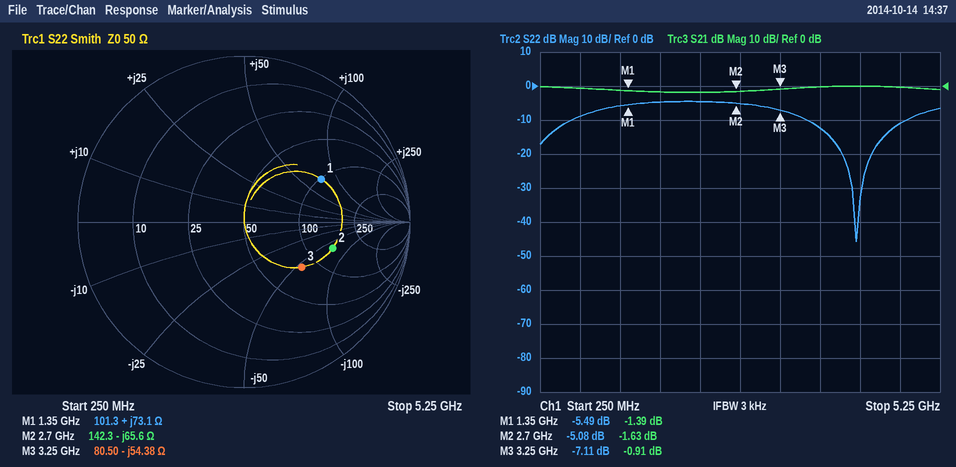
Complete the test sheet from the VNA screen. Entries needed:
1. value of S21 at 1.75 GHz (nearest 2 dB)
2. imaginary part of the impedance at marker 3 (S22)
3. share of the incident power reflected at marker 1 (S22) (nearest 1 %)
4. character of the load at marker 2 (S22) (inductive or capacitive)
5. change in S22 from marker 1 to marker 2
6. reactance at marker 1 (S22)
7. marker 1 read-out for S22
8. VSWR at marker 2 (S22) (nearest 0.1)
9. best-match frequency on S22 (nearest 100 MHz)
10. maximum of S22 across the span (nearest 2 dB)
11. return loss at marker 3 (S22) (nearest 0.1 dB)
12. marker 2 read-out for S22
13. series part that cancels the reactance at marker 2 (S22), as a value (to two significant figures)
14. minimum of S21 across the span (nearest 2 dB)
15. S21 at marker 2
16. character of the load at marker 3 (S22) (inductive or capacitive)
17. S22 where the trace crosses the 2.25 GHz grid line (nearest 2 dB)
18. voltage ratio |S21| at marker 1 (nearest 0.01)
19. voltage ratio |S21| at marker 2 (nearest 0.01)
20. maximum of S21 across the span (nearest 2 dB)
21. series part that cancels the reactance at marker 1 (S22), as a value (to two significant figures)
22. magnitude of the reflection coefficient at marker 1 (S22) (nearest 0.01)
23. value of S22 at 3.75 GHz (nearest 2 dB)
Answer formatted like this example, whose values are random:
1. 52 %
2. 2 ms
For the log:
1. -2 dB
2. -54.38 Ω
3. 28 %
4. capacitive
5. 0.41 dB
6. +73.1 Ω
7. -5.49 dB
8. 3.5
9. 4.2 GHz
10. -4 dB
11. 7.1 dB
12. -5.08 dB
13. 3.9 nH
14. -2 dB
15. -1.63 dB
16. capacitive
17. -4 dB
18. 0.85
19. 0.83
20. 0 dB
21. 1.6 pF
22. 0.53
23. -12 dB
